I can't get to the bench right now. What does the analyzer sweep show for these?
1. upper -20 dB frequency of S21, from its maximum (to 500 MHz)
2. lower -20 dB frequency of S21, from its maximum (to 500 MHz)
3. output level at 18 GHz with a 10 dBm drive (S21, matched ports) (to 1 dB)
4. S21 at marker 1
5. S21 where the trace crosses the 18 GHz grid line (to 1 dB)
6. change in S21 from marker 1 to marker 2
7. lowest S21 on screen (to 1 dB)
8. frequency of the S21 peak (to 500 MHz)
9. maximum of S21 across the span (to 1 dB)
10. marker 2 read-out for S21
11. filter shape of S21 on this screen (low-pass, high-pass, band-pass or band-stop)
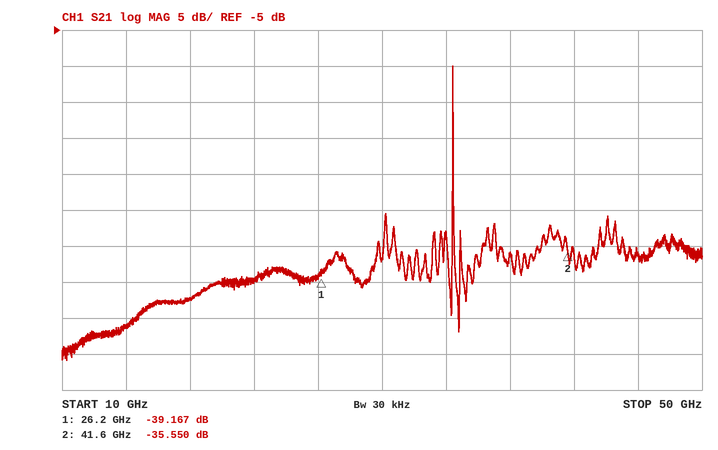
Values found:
34.5 GHz
34.5 GHz
-32 dBm
-39.167 dB
-42 dB
3.617 dB
-51 dB
34.5 GHz
-10 dB
-35.550 dB
band-pass
